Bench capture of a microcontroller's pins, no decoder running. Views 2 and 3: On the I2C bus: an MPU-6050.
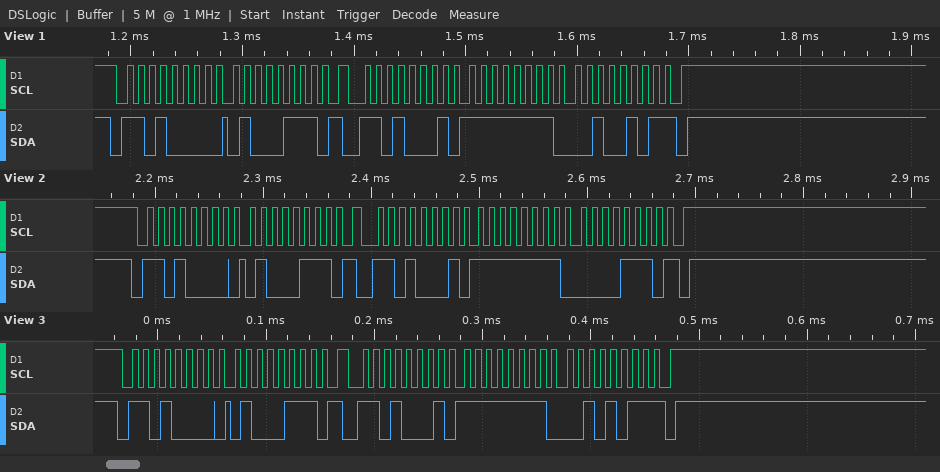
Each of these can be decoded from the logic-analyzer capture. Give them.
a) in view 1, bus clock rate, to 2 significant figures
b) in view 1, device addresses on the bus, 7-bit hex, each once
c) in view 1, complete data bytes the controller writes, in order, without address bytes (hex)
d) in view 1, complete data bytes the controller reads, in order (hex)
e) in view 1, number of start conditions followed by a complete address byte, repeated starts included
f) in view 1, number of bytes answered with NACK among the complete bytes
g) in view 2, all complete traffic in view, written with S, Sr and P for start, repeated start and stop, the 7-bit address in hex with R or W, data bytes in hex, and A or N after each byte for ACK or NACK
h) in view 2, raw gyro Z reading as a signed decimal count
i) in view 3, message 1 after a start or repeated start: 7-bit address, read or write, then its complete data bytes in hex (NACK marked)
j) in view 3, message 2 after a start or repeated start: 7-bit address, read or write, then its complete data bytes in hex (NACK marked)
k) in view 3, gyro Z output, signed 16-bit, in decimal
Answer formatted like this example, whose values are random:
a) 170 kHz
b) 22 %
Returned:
a) 100 kHz
b) 0x68
c) 47
d) FF 25
e) 2
f) 1
g) S 68W A 47 A Sr 68R A FF A 0E N P
h) -242
i) 0x68 write: 47
j) 0x68 read: FF 2B NACK
k) -213
